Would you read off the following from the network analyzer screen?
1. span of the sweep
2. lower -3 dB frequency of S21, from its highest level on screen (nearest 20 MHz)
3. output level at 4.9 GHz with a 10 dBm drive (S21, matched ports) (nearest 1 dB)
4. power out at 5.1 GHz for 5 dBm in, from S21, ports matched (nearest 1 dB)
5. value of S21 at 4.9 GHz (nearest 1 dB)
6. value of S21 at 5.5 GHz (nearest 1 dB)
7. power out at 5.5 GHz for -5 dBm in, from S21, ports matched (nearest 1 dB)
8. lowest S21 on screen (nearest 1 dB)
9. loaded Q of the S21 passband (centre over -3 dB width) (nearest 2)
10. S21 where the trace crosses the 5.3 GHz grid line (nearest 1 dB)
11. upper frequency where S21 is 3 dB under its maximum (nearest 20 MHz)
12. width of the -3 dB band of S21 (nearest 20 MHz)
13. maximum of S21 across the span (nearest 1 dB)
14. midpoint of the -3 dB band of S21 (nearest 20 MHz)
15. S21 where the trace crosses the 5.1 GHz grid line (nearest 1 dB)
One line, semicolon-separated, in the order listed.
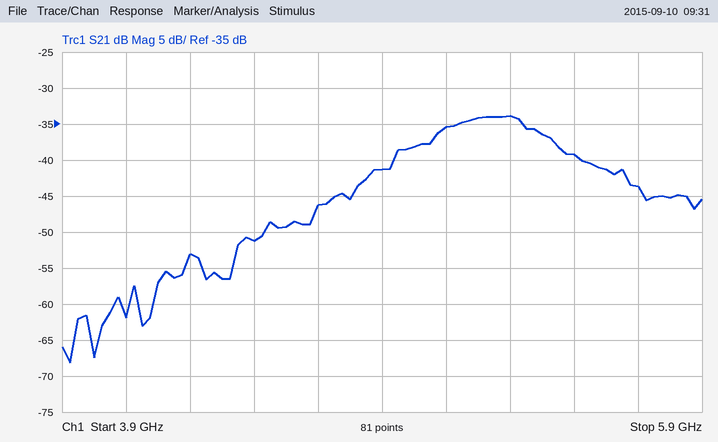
2 GHz; 5.06 GHz; -31 dBm; -30 dBm; -41 dB; -39 dB; -44 dBm; -68 dB; 14; -34 dB; 5.42 GHz; 360 MHz; -34 dB; 5.24 GHz; -35 dB
